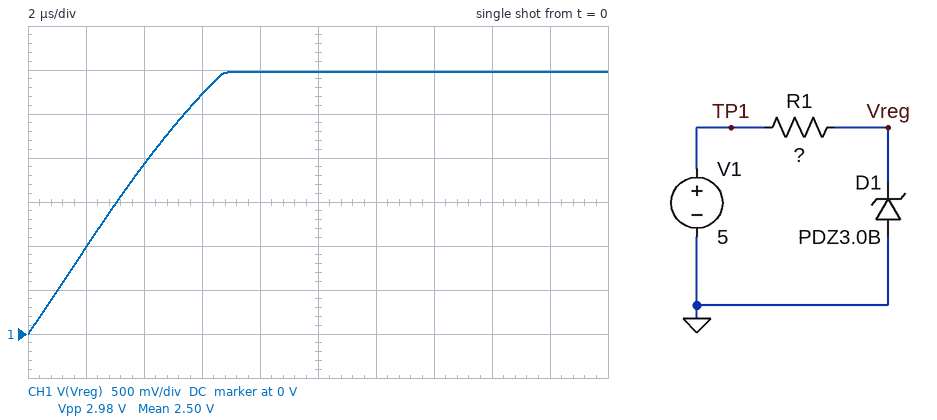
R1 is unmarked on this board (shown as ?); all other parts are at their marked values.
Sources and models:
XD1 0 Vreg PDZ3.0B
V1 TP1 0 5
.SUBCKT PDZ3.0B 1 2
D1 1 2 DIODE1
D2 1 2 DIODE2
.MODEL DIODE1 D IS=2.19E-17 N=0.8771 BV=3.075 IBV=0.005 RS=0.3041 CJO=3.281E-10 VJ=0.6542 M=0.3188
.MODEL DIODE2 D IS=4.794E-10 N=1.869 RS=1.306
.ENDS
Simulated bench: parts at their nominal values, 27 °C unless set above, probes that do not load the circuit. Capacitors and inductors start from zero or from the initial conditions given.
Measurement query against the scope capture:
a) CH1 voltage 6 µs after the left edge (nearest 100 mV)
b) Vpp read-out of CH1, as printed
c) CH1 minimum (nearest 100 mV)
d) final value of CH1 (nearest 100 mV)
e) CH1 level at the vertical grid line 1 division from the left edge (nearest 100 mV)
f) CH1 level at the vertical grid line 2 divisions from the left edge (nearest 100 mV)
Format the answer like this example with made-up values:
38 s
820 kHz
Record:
2.7 V
2.98 V
0 V
3.0 V
1.0 V
1.9 V
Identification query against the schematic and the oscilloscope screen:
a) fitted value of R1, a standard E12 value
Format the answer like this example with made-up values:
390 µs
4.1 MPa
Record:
33 kΩ
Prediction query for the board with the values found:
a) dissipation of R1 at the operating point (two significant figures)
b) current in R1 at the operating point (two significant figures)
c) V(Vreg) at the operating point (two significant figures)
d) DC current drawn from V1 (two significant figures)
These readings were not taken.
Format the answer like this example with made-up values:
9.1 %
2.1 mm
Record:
120 µW
61 µA
3.0 V
61 µA
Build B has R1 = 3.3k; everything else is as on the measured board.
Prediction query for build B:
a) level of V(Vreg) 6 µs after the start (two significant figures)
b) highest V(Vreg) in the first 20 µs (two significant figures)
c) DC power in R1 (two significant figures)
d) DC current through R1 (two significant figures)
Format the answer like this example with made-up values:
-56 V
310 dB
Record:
3.0 V
3.0 V
1.2 mW
600 µA
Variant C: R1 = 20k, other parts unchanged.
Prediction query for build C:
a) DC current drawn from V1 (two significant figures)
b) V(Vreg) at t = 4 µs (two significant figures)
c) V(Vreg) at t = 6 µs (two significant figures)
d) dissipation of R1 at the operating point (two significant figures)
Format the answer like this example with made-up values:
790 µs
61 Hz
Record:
100 µA
2.9 V
3.0 V
200 µW
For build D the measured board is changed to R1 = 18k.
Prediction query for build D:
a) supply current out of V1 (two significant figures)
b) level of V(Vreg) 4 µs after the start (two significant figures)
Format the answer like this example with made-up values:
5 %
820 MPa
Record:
110 µA
3.0 V
